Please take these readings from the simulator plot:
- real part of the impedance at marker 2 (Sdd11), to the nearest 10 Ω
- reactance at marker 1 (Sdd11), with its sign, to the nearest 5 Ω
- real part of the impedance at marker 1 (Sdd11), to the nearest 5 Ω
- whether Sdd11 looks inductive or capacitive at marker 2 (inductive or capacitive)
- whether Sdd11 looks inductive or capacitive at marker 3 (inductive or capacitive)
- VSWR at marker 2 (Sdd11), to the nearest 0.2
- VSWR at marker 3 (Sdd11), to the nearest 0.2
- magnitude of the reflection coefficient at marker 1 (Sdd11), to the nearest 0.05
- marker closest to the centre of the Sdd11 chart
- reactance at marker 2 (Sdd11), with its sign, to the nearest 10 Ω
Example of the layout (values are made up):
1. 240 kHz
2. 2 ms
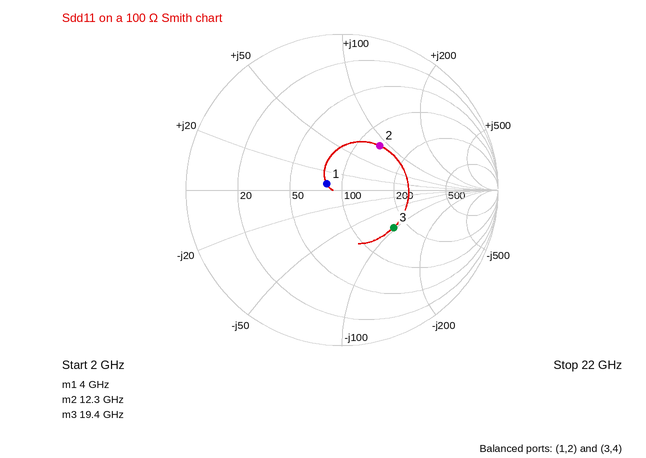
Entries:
1. 130 Ω
2. +5 Ω
3. 80 Ω
4. inductive
5. capacitive
6. 2.2
7. 2.4
8. 0.10
9. marker 1
10. +90 Ω
